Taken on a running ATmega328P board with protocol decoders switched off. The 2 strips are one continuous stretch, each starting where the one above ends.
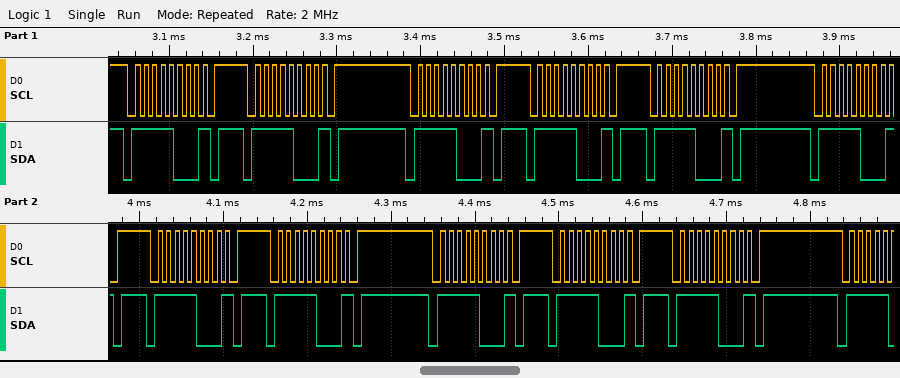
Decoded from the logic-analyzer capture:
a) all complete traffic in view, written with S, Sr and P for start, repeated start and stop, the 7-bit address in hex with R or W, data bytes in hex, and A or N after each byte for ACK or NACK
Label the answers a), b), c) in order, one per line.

a) S 7CW N P S 7CW N P S 7CW N P S 7CW N P S 7CW N P S 7CW N P S 7CW N P S 7CW N P S 7CW N P S 7CW N P S 7CW N P
